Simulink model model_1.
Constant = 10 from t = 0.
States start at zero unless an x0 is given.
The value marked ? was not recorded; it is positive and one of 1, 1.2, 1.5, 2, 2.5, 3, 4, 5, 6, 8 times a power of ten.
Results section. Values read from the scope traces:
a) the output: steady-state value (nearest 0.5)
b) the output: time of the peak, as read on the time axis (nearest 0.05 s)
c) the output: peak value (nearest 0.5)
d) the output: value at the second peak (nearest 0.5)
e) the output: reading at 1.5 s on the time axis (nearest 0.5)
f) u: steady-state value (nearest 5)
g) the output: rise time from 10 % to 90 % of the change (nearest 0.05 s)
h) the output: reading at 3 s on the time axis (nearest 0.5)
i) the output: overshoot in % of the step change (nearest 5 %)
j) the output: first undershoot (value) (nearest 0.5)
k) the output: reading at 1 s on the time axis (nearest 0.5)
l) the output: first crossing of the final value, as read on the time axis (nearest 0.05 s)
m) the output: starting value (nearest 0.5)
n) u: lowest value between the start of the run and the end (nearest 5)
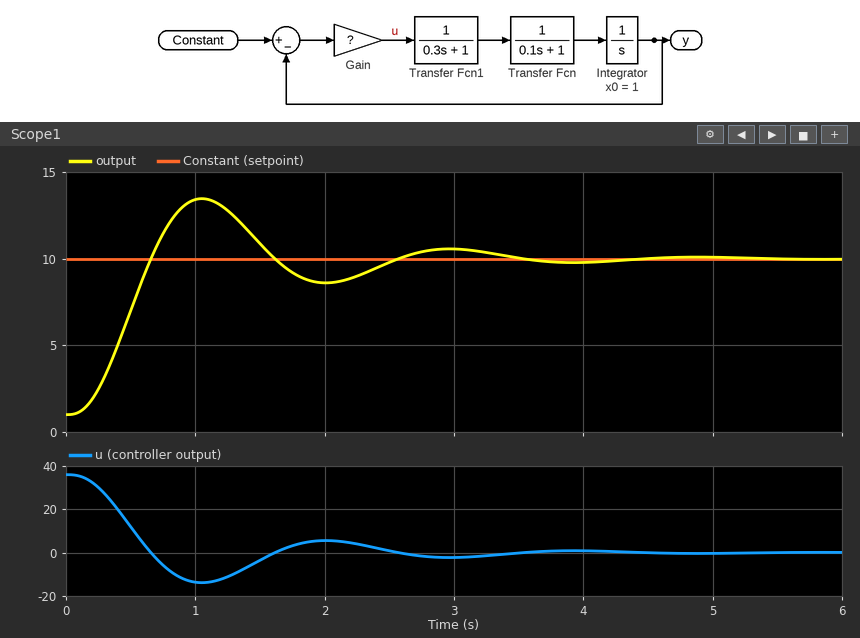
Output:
10.0
1.05 s
13.5
10.5
11.0
0
0.40 s
10.5
40 %
8.5
13.5
0.65 s
1.0
-15
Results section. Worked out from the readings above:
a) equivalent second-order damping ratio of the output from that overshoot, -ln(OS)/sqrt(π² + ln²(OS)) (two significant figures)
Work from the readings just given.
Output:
0.28
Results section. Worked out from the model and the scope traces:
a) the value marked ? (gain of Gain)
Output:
4
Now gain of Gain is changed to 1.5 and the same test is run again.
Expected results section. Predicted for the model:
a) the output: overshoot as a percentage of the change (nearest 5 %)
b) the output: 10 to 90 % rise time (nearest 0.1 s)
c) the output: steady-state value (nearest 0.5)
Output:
10 %
0.9 s
10.0
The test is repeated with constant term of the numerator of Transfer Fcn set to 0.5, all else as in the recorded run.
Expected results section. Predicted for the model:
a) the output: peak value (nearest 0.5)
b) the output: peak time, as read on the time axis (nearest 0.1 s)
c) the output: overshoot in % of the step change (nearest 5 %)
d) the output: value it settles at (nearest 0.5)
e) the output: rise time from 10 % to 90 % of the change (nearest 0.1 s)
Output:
11.5
1.6 s
15 %
10.0
0.7 s
